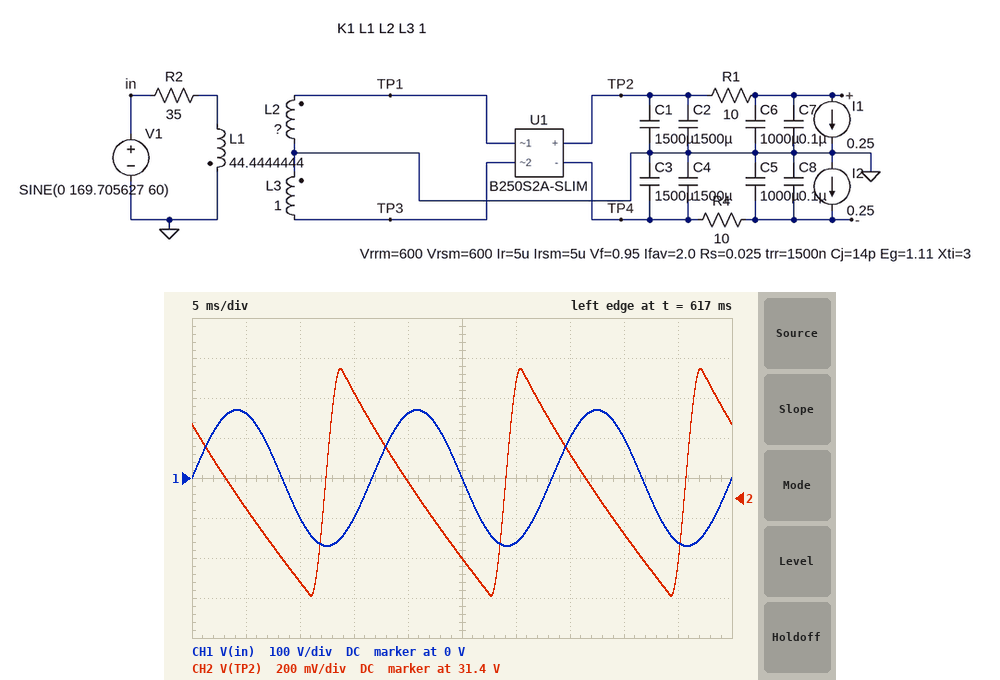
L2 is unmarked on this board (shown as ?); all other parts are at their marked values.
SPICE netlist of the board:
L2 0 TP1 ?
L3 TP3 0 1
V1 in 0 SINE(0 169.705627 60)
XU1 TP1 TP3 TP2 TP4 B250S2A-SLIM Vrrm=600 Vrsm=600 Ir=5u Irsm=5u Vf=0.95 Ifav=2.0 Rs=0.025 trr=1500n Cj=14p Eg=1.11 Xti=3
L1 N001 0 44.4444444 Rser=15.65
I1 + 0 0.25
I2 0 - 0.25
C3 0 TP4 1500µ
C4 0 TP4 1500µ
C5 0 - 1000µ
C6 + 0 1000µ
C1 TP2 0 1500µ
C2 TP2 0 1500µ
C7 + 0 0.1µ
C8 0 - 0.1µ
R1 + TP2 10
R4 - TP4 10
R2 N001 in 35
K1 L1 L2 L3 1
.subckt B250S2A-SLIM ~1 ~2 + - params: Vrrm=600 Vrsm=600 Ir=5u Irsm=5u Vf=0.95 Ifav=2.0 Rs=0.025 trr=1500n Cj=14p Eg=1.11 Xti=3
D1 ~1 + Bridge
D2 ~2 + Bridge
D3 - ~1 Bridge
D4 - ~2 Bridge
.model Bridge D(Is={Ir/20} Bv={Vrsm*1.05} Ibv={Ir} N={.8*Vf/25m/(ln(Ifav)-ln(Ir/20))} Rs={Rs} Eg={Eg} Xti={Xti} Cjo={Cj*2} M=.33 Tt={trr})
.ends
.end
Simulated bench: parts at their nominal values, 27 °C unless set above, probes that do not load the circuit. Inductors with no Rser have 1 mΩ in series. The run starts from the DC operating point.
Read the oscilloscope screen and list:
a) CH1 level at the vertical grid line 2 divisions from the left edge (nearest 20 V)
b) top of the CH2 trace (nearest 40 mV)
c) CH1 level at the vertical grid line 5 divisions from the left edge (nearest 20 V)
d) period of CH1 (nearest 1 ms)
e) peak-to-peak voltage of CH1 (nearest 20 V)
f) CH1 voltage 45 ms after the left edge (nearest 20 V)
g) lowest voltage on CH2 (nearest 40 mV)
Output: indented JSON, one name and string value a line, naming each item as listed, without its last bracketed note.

{
  "CH1 level at the vertical grid line 2 divisions from the left edge": "-100 V",
  "top of the CH2 trace": "32.04 V",
  "CH1 level at the vertical grid line 5 divisions from the left edge": "0 V",
  "period of CH1": "17 ms",
  "peak-to-peak voltage of CH1": "340 V",
  "CH1 voltage 45 ms after the left edge": "-160 V",
  "lowest voltage on CH2": "30.92 V"
}
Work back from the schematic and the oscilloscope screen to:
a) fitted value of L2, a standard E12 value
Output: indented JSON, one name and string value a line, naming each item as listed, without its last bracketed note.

{
  "fitted value of L2, a standard E12 value": "2.2 H"
}
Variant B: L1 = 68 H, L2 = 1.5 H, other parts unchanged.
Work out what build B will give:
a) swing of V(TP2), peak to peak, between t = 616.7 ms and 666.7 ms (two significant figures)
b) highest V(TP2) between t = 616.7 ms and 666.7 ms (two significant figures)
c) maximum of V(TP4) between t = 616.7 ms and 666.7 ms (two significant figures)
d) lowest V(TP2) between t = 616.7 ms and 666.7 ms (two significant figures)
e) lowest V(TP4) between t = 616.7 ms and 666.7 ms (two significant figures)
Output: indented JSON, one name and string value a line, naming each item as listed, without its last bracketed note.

{
  "swing of V(TP2), peak to peak, between t = 616.7 ms and 666.7 ms": "1.2 V",
  "highest V(TP2) between t = 616.7 ms and 666.7 ms": "22 V",
  "maximum of V(TP4) between t = 616.7 ms and 666.7 ms": "-21 V",
  "lowest V(TP2) between t = 616.7 ms and 666.7 ms": "21 V",
  "lowest V(TP4) between t = 616.7 ms and 666.7 ms": "-22 V"
}
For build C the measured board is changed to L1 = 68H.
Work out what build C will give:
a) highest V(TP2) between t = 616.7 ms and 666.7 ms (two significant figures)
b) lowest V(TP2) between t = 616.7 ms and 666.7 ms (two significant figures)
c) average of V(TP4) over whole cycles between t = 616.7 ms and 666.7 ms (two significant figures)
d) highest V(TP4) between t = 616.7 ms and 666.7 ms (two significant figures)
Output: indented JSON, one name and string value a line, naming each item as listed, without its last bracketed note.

{
  "highest V(TP2) between t = 616.7 ms and 666.7 ms": "26 V",
  "lowest V(TP2) between t = 616.7 ms and 666.7 ms": "25 V",
  "average of V(TP4) over whole cycles between t = 616.7 ms and 666.7 ms": "-26 V",
  "highest V(TP4) between t = 616.7 ms and 666.7 ms": "-25 V"
}
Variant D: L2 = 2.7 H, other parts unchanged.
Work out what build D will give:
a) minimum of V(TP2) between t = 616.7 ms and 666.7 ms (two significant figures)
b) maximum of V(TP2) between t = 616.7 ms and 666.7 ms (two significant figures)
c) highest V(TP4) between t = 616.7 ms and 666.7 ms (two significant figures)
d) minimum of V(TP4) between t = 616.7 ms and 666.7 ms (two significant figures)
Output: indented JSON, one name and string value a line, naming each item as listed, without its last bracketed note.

{
  "minimum of V(TP2) between t = 616.7 ms and 666.7 ms": "34 V",
  "maximum of V(TP2) between t = 616.7 ms and 666.7 ms": "35 V",
  "highest V(TP4) between t = 616.7 ms and 666.7 ms": "-34 V",
  "minimum of V(TP4) between t = 616.7 ms and 666.7 ms": "-35 V"
}
